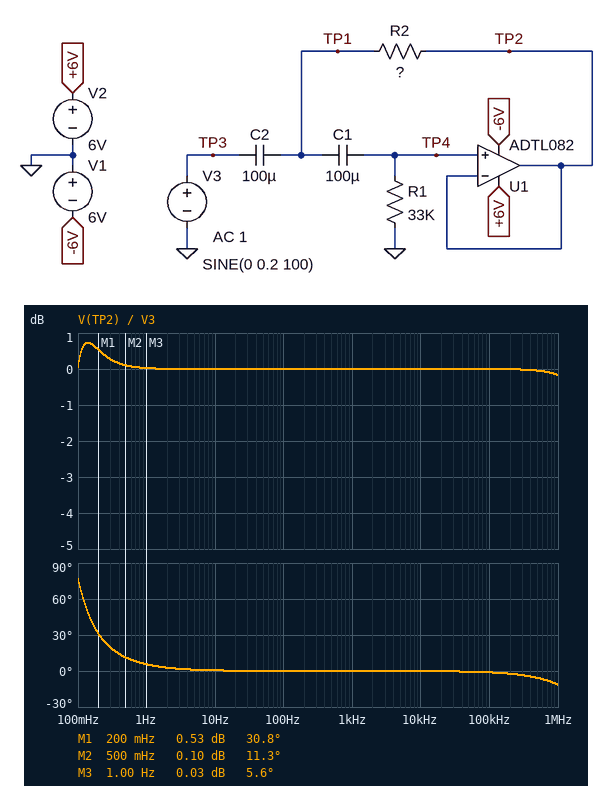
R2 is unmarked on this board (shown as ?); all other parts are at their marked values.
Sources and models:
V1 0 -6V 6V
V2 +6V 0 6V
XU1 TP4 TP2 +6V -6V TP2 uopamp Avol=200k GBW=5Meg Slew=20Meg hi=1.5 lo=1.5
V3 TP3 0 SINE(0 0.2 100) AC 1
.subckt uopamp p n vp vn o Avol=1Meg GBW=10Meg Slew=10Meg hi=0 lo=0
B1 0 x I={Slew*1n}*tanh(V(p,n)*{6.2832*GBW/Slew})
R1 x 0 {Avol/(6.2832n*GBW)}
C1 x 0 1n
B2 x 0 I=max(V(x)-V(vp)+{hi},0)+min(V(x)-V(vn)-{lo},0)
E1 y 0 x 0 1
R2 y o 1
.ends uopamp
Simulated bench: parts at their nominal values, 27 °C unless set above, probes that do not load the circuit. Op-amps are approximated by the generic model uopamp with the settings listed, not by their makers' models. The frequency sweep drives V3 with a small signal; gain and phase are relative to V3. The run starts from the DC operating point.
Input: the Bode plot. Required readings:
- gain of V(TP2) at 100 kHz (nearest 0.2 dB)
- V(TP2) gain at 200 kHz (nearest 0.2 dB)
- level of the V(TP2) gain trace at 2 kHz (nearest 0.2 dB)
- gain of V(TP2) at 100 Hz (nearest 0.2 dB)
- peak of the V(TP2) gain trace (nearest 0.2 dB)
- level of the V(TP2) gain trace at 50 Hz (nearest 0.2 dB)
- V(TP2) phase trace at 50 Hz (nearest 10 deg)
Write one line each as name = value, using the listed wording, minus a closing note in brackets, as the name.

gain of V(TP2) at 100 kHz = 0 dB
V(TP2) gain at 200 kHz = 0 dB
level of the V(TP2) gain trace at 2 kHz = 0 dB
gain of V(TP2) at 100 Hz = 0 dB
peak of the V(TP2) gain trace = 0.8 dB
level of the V(TP2) gain trace at 50 Hz = 0 dB
V(TP2) phase trace at 50 Hz = 0 deg
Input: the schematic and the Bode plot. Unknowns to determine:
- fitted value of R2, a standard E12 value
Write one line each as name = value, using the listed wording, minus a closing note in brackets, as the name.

fitted value of R2, a standard E12 value = 10 kΩ
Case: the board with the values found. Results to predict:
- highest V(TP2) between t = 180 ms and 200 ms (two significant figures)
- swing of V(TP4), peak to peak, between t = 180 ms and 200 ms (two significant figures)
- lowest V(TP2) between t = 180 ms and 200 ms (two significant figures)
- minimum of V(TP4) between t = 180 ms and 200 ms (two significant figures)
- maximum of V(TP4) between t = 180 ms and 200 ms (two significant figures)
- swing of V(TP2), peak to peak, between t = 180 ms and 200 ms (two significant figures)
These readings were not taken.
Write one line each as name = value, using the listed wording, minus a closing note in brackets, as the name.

highest V(TP2) between t = 180 ms and 200 ms = 200 mV
swing of V(TP4), peak to peak, between t = 180 ms and 200 ms = 400 mV
lowest V(TP2) between t = 180 ms and 200 ms = -200 mV
minimum of V(TP4) between t = 180 ms and 200 ms = -200 mV
maximum of V(TP4) between t = 180 ms and 200 ms = 200 mV
swing of V(TP2), peak to peak, between t = 180 ms and 200 ms = 400 mV
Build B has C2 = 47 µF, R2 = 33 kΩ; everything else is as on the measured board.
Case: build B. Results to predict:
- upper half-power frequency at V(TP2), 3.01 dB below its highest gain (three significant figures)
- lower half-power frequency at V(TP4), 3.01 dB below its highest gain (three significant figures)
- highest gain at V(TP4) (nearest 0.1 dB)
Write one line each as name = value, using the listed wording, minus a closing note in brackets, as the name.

upper half-power frequency at V(TP2), 3.01 dB below its highest gain = 5.00 MHz
lower half-power frequency at V(TP4), 3.01 dB below its highest gain = 121 mHz
highest gain at V(TP4) = 0 dB
